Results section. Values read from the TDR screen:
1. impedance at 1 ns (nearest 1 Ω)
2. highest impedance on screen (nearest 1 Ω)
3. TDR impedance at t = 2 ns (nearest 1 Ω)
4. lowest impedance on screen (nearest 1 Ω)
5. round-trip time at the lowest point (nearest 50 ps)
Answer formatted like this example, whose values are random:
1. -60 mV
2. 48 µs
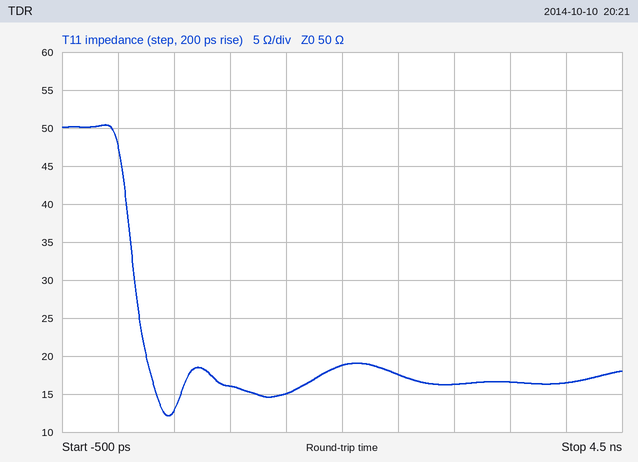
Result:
1. 16 Ω
2. 50 Ω
3. 19 Ω
4. 12 Ω
5. 450 ps
